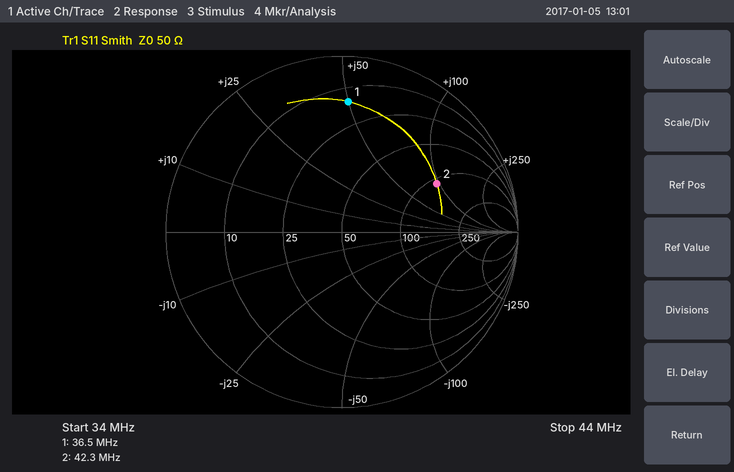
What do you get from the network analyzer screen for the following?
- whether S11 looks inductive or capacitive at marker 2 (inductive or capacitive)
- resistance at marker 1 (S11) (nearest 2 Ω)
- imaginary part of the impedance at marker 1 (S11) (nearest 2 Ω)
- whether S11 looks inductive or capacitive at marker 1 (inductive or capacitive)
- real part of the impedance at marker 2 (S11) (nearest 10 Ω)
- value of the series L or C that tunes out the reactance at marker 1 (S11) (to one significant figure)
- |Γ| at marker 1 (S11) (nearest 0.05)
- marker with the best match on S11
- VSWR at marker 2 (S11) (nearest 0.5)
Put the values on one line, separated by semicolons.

inductive; 16 Ω; +50 Ω; inductive; 110 Ω; 90 pF; 0.75; marker 2; 4.0
